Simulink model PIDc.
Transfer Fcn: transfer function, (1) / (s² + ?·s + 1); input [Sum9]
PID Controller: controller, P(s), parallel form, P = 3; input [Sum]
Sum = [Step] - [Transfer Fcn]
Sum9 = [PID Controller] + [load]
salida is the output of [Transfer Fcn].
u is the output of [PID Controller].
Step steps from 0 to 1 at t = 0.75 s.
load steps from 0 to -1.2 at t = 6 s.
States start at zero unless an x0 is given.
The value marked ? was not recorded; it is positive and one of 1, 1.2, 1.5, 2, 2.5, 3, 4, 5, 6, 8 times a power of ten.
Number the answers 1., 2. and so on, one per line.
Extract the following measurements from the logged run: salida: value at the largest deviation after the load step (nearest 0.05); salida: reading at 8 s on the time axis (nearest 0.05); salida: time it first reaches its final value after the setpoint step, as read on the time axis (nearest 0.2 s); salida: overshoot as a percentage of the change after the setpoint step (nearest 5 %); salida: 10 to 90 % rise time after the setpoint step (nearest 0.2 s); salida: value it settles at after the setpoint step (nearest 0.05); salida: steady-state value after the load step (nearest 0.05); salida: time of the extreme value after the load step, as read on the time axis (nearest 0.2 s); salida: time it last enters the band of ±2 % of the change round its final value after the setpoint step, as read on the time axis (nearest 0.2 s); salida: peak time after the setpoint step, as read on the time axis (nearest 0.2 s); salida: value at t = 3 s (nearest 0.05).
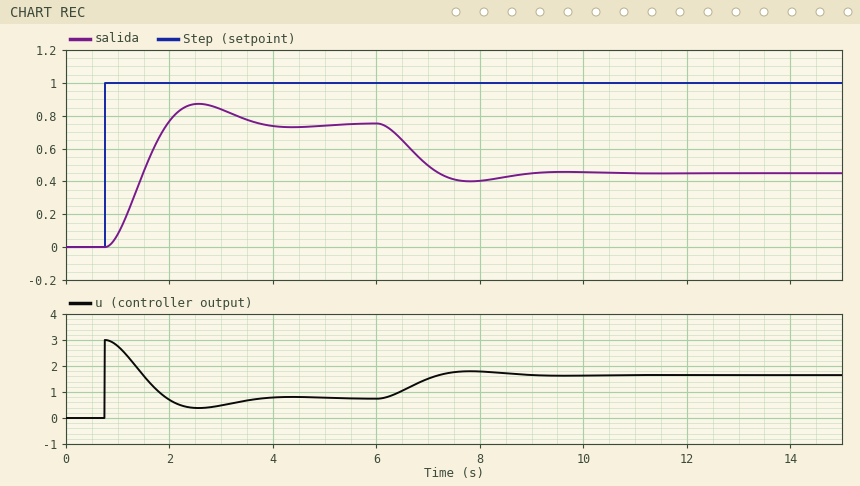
1. 0.40
2. 0.40
3. 2.0 s
4. 15 %
5. 0.8 s
6. 0.75
7. 0.45
8. 7.8 s
9. 4.8 s
10. 2.6 s
11. 0.85
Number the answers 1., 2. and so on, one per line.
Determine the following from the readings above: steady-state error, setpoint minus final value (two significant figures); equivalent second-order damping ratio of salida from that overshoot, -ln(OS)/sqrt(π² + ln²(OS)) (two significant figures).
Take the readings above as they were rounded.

1. 0.25
2. 0.52
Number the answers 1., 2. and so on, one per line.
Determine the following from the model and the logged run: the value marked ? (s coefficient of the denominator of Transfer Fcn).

1. 2
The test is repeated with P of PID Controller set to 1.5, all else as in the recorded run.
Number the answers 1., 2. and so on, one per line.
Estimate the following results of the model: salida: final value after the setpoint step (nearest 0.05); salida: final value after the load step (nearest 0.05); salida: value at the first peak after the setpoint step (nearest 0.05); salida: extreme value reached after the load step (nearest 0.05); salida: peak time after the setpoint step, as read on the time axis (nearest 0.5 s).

1. 0.60
2. 0.10
3. 0.65
4. 0.10
5. 3.5 s
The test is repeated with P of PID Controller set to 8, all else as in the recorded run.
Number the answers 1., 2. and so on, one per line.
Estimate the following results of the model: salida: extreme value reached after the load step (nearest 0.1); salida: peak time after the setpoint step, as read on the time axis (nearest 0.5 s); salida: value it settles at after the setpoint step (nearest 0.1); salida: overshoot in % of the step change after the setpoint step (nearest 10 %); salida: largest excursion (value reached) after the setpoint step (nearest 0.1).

1. 0.7
2. 2.0 s
3. 0.9
4. 30 %
5. 1.2
